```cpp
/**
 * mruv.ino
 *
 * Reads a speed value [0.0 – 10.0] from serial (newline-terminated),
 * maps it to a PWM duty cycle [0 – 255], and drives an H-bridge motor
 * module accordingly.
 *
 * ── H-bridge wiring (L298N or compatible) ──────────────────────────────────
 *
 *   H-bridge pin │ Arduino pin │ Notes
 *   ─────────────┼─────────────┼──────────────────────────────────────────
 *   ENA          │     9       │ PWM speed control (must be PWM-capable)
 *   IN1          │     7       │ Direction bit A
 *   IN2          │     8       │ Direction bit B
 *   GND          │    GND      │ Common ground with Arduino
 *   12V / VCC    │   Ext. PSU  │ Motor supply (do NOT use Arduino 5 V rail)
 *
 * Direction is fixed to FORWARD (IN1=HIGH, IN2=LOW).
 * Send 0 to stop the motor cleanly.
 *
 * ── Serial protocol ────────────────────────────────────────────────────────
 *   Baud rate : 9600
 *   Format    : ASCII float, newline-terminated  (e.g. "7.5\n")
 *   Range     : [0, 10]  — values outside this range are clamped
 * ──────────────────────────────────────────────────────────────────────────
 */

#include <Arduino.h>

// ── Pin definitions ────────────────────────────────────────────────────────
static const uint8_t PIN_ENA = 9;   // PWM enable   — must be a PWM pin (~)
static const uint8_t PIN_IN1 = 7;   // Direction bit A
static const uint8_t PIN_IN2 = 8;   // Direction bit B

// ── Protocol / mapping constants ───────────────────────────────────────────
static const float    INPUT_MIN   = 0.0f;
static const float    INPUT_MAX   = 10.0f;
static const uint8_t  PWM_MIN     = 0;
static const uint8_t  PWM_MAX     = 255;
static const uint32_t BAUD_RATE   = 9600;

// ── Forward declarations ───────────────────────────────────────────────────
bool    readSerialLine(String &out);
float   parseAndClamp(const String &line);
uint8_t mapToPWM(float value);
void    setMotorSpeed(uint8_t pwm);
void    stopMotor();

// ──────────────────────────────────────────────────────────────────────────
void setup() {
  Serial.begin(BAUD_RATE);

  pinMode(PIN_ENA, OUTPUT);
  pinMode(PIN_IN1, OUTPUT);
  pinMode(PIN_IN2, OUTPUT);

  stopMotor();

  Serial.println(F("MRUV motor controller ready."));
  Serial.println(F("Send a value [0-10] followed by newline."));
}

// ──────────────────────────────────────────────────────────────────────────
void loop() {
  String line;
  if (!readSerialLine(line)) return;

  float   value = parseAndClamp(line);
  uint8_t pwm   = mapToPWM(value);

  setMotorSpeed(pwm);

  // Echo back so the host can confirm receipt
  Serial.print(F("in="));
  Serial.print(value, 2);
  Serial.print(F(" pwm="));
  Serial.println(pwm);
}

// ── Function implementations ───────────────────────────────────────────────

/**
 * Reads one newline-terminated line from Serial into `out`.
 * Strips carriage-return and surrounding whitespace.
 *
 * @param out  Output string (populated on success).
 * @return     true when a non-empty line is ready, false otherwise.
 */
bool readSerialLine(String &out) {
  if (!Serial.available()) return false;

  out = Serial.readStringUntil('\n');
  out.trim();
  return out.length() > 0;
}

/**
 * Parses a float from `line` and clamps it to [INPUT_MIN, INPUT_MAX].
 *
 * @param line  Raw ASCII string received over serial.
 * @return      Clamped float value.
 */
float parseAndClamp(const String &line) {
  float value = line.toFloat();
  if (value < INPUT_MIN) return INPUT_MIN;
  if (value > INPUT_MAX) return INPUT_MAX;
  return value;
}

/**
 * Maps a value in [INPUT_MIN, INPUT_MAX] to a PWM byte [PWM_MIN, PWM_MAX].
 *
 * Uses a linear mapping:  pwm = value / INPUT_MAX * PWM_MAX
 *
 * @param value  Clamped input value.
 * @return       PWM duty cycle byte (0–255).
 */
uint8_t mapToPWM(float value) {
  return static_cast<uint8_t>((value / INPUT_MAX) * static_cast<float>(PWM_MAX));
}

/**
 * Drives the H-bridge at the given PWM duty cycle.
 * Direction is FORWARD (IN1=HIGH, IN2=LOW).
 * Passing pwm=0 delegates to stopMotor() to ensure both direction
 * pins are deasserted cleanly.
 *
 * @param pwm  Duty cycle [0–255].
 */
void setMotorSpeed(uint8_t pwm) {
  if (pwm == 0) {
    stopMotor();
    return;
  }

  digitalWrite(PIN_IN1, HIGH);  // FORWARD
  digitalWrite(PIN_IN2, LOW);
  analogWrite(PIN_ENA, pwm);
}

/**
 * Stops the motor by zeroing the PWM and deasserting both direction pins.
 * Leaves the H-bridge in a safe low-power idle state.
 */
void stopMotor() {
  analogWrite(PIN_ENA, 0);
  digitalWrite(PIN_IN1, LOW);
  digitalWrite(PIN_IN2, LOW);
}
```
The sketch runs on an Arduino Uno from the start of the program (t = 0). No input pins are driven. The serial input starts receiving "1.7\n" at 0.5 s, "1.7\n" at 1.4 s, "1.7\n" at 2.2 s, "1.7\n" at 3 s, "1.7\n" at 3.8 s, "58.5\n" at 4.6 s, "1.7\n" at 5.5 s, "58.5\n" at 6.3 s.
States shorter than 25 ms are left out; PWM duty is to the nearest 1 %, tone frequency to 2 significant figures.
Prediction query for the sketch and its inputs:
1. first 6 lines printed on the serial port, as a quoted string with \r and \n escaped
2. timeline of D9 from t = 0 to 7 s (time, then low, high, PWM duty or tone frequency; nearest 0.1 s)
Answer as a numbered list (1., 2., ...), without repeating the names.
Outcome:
1. "MRUV motor controller ready.\r\nSend a value [0-10] followed by newline.\r\nin=1.70 pwm=43\r\nin=1.70 pwm=43\r\nin=1.70 pwm=43\r\nin=1.70 pwm=43\r\n"
2. 0 s low; 0.5 s PWM 17 %; 4.6 s high; 5.5 s PWM 17 %; 6.3 s high
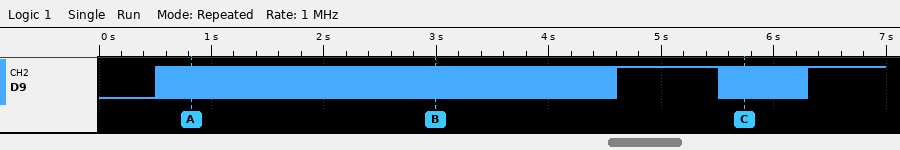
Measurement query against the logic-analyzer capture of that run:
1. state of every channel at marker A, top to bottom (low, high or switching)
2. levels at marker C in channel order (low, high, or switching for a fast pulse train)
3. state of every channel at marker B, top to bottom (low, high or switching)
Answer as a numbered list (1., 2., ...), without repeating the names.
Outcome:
1. D9 switching
2. D9 switching
3. D9 switching
